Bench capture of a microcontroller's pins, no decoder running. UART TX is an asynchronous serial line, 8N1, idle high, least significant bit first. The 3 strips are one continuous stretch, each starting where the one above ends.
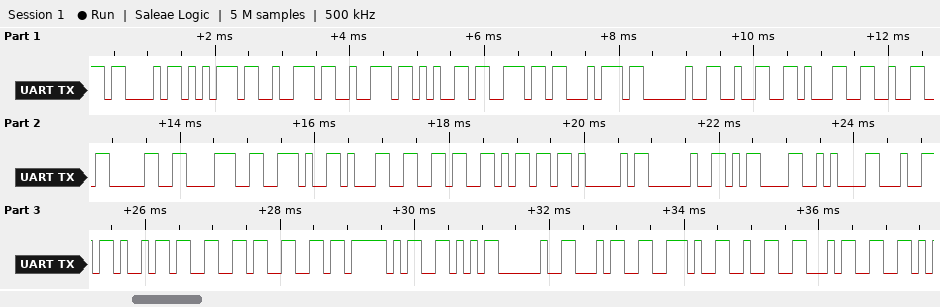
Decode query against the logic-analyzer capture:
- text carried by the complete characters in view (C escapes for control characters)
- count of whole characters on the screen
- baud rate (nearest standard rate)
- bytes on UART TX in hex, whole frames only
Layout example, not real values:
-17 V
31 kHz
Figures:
"Current 21208.16mA \r\ndiff_V 4.24"
32
9600 baud
0x43 0x75 0x72 0x72 0x65 0x6E 0x74 0x20 0x32 0x31 0x32 0x30 0x38 0x2E 0x31 0x36 0x6D 0x41 0x20 0x0D 0x0A 0x64 0x69 0x66 0x66 0x5F 0x56 0x20 0x34 0x2E 0x32 0x34
